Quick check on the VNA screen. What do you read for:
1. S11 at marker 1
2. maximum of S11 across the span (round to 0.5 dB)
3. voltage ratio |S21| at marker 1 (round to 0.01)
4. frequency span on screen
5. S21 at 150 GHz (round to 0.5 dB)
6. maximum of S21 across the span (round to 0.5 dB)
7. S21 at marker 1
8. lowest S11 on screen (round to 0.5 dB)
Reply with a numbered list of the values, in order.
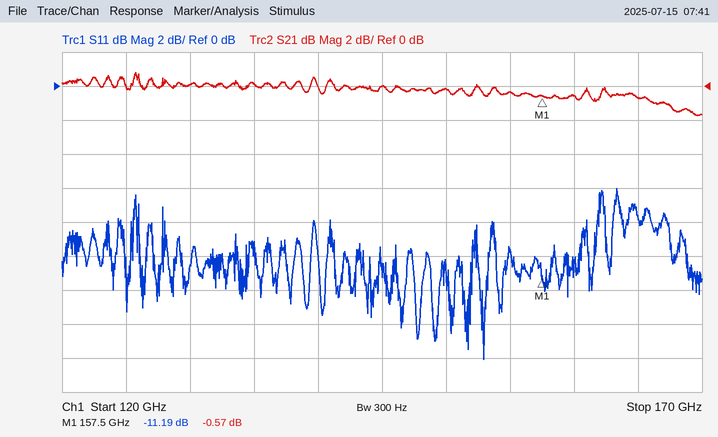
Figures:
1. -11.19 dB
2. -6.0 dB
3. 0.94
4. 50 GHz
5. 0.0 dB
6. 1.0 dB
7. -0.57 dB
8. -16.0 dB
